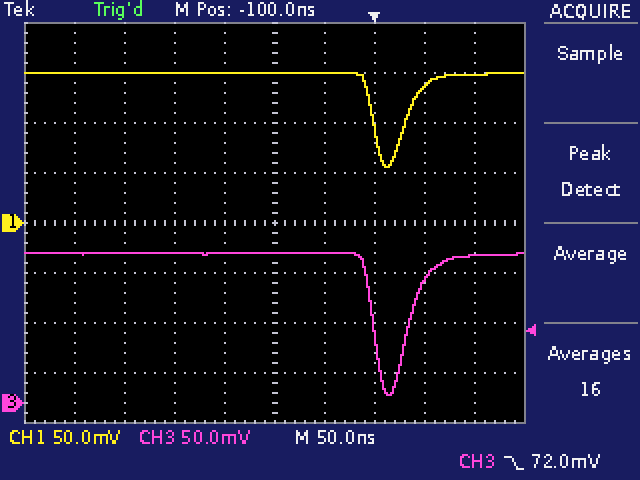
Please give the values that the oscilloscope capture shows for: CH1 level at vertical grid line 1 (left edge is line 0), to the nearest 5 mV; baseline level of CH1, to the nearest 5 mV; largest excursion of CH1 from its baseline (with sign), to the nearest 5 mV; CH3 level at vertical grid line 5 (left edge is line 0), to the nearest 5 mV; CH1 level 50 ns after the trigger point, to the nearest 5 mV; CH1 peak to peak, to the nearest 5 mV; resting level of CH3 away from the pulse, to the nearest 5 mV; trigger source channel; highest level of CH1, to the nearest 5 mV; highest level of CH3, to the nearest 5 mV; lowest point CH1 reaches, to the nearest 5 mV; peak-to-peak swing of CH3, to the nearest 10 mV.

150 mV
150 mV
-95 mV
150 mV
135 mV
95 mV
150 mV
CH3
150 mV
150 mV
55 mV
140 mV
